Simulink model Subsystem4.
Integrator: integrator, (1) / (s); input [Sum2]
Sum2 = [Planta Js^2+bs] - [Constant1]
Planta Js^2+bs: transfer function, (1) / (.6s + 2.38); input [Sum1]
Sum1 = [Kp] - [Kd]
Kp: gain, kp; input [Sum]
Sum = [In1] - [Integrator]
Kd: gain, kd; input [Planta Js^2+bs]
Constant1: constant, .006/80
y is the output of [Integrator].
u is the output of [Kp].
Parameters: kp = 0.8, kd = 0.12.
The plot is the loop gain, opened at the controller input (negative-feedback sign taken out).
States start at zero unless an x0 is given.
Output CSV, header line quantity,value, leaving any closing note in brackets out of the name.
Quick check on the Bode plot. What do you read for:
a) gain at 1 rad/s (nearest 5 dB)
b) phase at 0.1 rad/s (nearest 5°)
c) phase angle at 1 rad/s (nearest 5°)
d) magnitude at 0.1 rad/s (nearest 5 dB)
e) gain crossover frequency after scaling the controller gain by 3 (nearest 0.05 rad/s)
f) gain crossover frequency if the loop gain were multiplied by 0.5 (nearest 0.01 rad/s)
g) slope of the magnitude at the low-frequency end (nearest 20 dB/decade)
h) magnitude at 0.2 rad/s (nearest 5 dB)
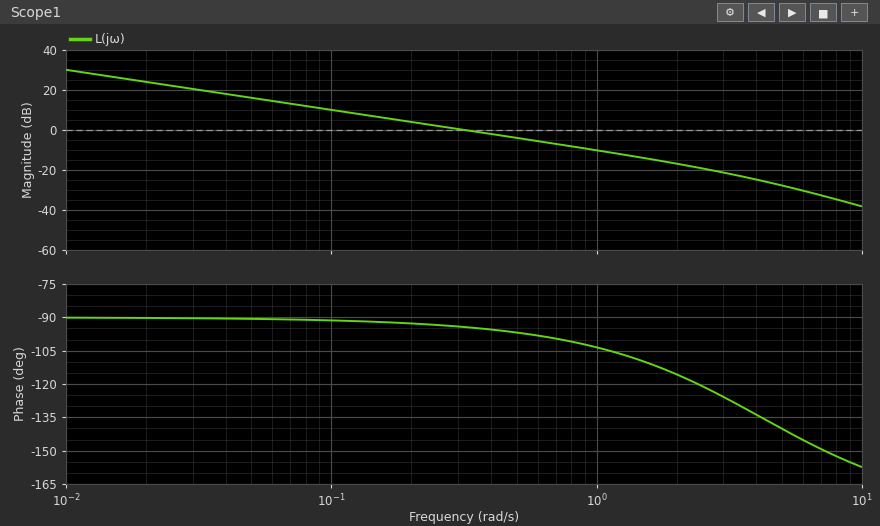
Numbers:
quantity,value
gain at 1 rad/s,-10 dB
phase at 0.1 rad/s,-90°
phase angle at 1 rad/s,-105°
magnitude at 0.1 rad/s,10 dB
gain crossover frequency after scaling the controller gain by 3,0.95 rad/s
gain crossover frequency if the loop gain were multiplied by 0.5,0.16 rad/s
slope of the magnitude at the low-frequency end,-20 dB/decade
magnitude at 0.2 rad/s,5 dB
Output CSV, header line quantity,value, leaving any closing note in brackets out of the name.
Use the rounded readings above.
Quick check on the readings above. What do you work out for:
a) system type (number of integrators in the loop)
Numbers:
quantity,value
system type,1
